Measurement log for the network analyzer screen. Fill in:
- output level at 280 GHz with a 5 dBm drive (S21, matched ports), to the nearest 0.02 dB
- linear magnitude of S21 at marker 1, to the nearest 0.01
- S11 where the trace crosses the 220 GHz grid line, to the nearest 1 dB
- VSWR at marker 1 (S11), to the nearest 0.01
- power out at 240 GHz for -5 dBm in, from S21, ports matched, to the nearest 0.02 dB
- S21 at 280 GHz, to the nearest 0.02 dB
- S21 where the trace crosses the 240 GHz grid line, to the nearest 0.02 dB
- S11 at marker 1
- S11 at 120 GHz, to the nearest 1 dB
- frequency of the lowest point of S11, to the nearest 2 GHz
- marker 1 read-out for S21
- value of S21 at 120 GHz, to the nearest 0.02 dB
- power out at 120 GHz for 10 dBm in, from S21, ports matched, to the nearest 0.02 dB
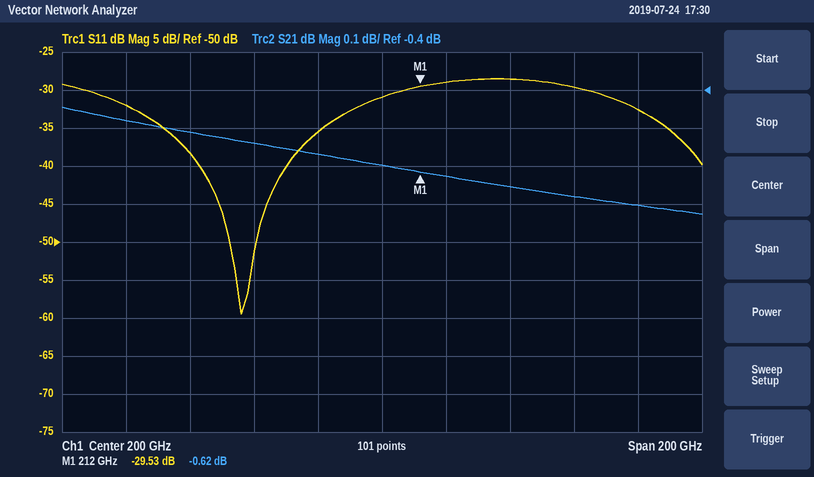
4.30 dBm
0.93
-29 dB
1.07
-5.66 dBm
-0.70 dB
-0.66 dB
-29.53 dB
-32 dB
156 GHz
-0.62 dB
-0.48 dB
9.52 dBm
